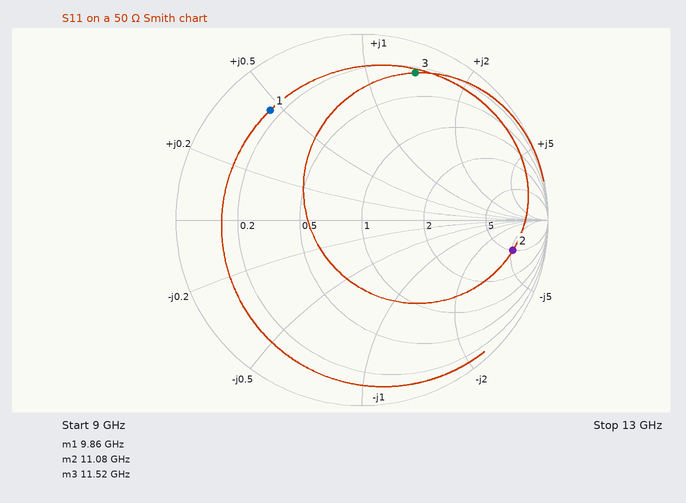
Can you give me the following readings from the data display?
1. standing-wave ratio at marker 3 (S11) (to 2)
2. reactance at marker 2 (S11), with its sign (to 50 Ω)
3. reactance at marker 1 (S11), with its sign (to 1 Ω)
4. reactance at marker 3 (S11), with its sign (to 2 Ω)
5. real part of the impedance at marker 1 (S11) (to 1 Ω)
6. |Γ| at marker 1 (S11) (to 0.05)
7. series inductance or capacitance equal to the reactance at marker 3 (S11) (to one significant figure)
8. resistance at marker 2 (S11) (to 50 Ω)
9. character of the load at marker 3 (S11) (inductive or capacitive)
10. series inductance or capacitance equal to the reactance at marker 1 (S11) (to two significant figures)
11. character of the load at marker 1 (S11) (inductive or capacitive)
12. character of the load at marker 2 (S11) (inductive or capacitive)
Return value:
12
-250 Ω
+23 Ω
+70 Ω
8 Ω
0.75
1.0 nH
250 Ω
inductive
370 pH
inductive
capacitive
